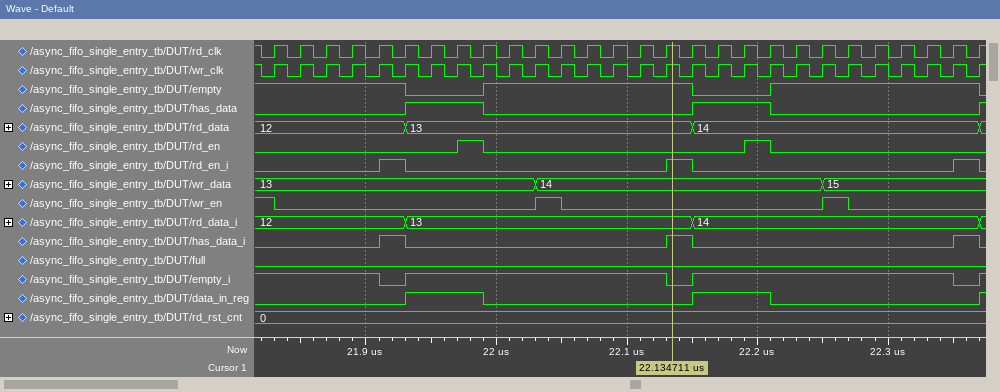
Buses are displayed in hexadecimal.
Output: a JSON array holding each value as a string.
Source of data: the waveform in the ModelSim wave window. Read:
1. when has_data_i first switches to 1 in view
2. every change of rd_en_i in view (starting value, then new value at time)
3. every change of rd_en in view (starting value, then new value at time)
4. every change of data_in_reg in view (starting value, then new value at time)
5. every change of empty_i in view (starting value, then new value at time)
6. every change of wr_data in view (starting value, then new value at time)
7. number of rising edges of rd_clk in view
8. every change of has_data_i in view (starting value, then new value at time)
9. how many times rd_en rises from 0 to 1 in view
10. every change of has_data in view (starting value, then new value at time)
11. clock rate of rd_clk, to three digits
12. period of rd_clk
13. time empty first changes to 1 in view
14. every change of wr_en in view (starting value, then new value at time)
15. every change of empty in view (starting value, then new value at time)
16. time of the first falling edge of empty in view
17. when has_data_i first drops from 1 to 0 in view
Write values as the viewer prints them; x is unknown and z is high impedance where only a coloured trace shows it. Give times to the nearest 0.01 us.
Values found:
["21.91 us", "0, 1 at 21.91 us, 0 at 21.93 us, 1 at 22.13 us, 0 at 22.15 us, 1 at 22.35 us, 0 at 22.37 us", "0, 1 at 21.97 us, 0 at 21.99 us, 1 at 22.19 us, 0 at 22.21 us", "0, 1 at 21.93 us, 0 at 21.99 us, 1 at 22.15 us, 0 at 22.21 us, 1 at 22.37 us", "1, 0 at 21.91 us, 1 at 21.93 us, 0 at 22.13 us, 1 at 22.15 us, 0 at 22.35 us, 1 at 22.37 us", "13, 14 at 22.03 us, 15 at 22.25 us", "28", "0, 1 at 21.91 us, 0 at 21.93 us, 1 at 22.13 us, 0 at 22.15 us, 1 at 22.35 us, 0 at 22.37 us", "2", "0, 1 at 21.93 us, 0 at 21.99 us, 1 at 22.15 us, 0 at 22.21 us, 1 at 22.37 us", "50.0 MHz", "0.02 us", "21.99 us", "1, 0 at 21.83 us, 1 at 22.03 us, 0 at 22.05 us, 1 at 22.25 us, 0 at 22.27 us", "1, 0 at 21.93 us, 1 at 21.99 us, 0 at 22.15 us, 1 at 22.21 us, 0 at 22.37 us", "21.93 us", "21.93 us"]
